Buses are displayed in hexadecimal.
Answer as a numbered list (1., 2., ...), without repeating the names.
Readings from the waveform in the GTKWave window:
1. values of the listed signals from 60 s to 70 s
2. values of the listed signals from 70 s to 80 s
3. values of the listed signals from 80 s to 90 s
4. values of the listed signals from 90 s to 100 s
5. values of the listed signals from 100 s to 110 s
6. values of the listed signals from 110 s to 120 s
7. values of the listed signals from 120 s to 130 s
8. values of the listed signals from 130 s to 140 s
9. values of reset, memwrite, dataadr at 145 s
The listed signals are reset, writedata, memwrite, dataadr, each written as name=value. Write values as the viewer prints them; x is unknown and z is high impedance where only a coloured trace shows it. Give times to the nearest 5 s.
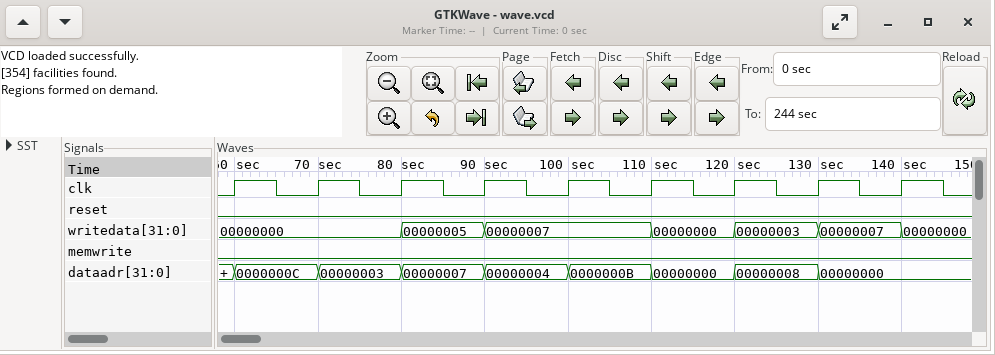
1. reset=0, writedata=00000000, memwrite=0, dataadr=0000000C
2. reset=0, writedata=00000000, memwrite=0, dataadr=00000003
3. reset=0, writedata=00000005, memwrite=0, dataadr=00000007
4. reset=0, writedata=00000007, memwrite=0, dataadr=00000004
5. reset=0, writedata=00000007, memwrite=0, dataadr=0000000B
6. reset=0, writedata=00000000, memwrite=0, dataadr=00000000
7. reset=0, writedata=00000003, memwrite=0, dataadr=00000008
8. reset=0, writedata=00000007, memwrite=0, dataadr=00000000
9. reset=0, memwrite=0, dataadr=00000000
